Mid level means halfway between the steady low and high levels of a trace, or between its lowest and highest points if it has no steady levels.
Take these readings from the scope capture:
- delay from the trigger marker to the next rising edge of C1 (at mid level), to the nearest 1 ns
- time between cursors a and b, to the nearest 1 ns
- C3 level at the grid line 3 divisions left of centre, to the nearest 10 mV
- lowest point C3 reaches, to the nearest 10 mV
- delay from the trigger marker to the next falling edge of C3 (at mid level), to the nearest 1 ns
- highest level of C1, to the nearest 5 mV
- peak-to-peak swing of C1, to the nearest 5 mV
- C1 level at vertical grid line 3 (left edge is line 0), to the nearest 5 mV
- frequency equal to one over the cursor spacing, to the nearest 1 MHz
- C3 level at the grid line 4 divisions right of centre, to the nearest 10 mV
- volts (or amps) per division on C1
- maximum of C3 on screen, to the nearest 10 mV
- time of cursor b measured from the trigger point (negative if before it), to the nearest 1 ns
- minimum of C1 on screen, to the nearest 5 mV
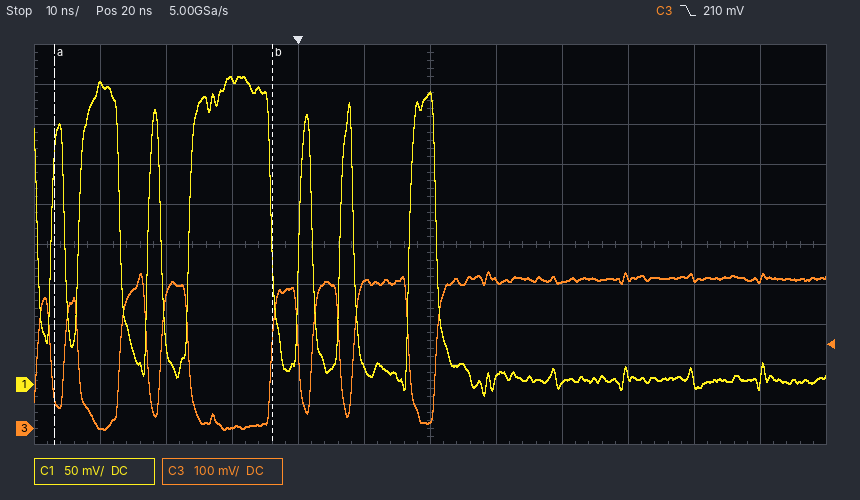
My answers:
6 ns
33 ns
0 mV
0 mV
6 ns
385 mV
400 mV
380 mV
30 MHz
380 mV
50 mV
390 mV
-4 ns
-15 mV
